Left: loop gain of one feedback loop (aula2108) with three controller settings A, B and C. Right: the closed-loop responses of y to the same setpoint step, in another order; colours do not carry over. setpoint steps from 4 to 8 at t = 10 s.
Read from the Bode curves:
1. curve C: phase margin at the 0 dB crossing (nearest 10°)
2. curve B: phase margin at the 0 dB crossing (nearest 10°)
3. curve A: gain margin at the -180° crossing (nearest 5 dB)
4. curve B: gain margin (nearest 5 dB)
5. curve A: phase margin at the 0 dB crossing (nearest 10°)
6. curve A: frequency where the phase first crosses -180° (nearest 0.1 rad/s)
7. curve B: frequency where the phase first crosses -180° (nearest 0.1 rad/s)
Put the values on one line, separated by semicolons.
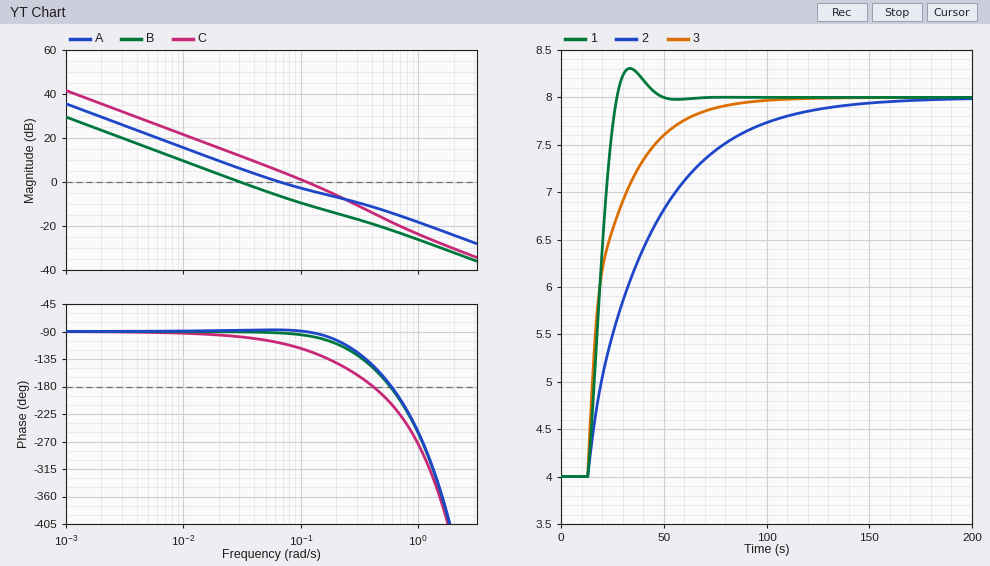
60°; 90°; 15 dB; 20 dB; 90°; 0.6 rad/s; 0.6 rad/s
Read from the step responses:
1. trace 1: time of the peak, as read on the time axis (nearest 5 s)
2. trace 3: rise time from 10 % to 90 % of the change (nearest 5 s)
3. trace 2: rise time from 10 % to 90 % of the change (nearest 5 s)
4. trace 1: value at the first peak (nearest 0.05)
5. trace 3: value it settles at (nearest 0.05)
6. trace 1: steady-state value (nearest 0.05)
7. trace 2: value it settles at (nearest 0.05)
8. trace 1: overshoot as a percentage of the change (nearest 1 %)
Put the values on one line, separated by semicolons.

35 s; 35 s; 70 s; 8.30; 8.00; 8.00; 8.00; 8 %
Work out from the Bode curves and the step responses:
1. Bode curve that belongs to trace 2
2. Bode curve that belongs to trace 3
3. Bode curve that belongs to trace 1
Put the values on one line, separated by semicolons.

B; A; C
